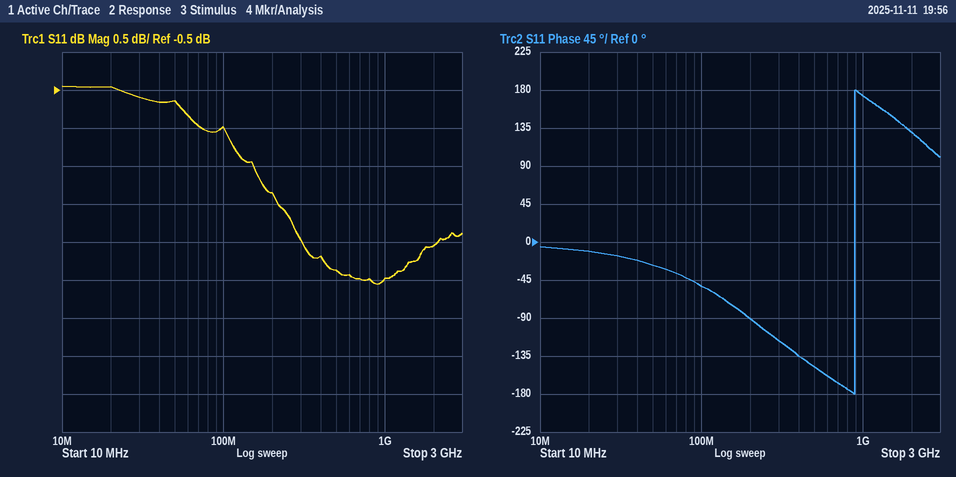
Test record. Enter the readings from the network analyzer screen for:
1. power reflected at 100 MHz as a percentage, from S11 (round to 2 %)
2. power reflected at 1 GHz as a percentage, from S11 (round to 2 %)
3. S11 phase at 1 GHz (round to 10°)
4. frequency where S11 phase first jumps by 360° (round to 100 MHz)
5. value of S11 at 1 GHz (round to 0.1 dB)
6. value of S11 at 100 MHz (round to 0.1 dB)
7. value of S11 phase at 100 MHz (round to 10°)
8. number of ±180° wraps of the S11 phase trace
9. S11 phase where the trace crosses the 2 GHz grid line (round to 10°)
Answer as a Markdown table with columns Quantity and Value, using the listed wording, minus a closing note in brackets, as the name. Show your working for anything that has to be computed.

| Quantity | Value |
|---|---|
| power reflected at 100 MHz as a percentage, from S11 | 10^(-1/10) ≈ 79.4 %, so 80 % to the nearest 2 % |
| power reflected at 1 GHz as a percentage, from S11 | 10^(-3/10) ≈ 50 % |
| S11 phase at 1 GHz | 170° |
| frequency where S11 phase first jumps by 360° | 900 MHz |
| value of S11 at 1 GHz | -3.0 dB |
| value of S11 at 100 MHz | -1.0 dB |
| value of S11 phase at 100 MHz | -50° |
| number of ±180° wraps of the S11 phase trace | 1 |
| S11 phase where the trace crosses the 2 GHz grid line | 130° |
